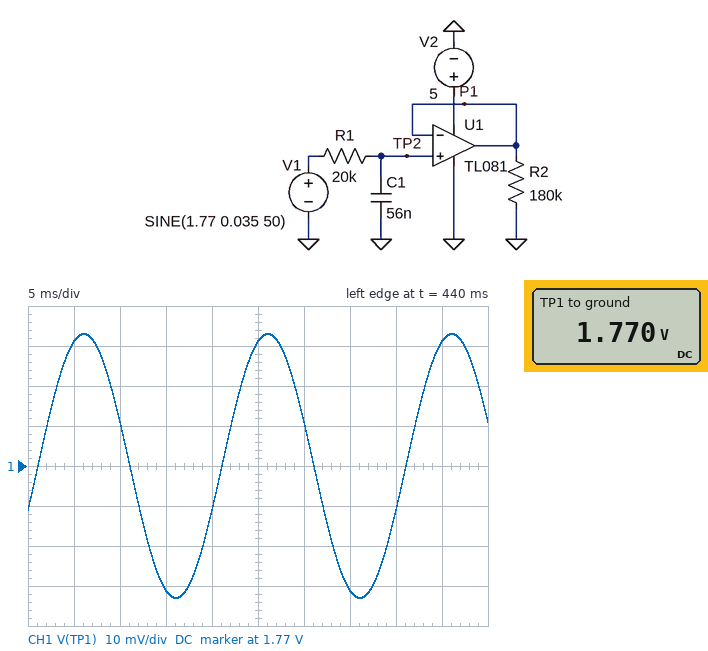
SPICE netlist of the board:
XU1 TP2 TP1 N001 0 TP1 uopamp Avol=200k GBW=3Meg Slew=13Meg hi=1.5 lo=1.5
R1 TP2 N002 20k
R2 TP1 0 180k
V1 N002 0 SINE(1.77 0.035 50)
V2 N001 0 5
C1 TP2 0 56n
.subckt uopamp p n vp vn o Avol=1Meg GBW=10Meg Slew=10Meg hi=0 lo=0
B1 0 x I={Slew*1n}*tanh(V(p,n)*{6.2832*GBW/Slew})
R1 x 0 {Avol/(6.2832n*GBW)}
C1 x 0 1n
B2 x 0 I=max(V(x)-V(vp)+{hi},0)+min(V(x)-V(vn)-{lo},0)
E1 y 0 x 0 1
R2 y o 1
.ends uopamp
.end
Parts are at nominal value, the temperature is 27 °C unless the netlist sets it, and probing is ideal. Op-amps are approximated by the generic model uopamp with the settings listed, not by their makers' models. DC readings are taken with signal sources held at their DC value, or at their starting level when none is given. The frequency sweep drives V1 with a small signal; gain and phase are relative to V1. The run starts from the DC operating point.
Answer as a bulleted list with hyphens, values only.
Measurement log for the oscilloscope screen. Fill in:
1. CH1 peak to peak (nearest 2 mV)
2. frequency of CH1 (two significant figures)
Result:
- 66 mV
- 50 Hz
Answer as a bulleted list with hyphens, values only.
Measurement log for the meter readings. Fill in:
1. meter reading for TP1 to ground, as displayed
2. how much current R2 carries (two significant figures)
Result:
- 1.770 V
- 9.8 µA
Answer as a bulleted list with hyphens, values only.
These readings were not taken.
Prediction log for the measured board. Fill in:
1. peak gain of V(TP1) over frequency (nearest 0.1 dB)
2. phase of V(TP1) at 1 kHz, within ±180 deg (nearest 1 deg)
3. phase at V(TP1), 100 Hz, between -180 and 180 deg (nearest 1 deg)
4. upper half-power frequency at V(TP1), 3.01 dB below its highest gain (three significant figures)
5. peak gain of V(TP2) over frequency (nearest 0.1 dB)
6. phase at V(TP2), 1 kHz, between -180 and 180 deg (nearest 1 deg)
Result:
- 0 dB
- -82 deg
- -35 deg
- 142 Hz
- 0 dB
- -82 deg
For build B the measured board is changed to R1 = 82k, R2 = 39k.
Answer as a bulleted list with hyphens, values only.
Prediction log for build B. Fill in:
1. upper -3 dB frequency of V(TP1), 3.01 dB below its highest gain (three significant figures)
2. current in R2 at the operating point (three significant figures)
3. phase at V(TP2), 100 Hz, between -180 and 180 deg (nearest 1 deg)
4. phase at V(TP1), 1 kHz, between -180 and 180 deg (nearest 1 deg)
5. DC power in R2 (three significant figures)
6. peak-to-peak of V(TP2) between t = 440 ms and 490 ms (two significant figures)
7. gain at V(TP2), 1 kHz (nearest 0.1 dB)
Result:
- 34.7 Hz
- 45.4 µA
- -71 deg
- -88 deg
- 80.3 µW
- 40 mV
- -29.2 dB
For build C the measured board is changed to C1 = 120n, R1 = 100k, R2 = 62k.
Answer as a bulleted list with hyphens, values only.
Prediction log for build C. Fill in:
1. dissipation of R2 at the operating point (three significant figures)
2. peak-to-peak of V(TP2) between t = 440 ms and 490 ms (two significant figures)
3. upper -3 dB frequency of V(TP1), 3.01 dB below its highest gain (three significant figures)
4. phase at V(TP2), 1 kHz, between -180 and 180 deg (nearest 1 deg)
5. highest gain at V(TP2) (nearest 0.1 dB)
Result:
- 50.5 µW
- 18 mV
- 13.3 Hz
- -89 deg
- 0 dB
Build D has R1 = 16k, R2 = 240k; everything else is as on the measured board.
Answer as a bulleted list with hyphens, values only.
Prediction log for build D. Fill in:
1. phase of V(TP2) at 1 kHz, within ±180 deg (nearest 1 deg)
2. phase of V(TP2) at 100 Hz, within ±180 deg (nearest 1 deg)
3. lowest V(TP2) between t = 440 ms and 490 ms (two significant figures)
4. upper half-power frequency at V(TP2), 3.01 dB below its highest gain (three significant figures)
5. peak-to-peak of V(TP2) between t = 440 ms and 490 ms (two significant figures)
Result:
- -80 deg
- -29 deg
- 1.7 V
- 178 Hz
- 67 mV
